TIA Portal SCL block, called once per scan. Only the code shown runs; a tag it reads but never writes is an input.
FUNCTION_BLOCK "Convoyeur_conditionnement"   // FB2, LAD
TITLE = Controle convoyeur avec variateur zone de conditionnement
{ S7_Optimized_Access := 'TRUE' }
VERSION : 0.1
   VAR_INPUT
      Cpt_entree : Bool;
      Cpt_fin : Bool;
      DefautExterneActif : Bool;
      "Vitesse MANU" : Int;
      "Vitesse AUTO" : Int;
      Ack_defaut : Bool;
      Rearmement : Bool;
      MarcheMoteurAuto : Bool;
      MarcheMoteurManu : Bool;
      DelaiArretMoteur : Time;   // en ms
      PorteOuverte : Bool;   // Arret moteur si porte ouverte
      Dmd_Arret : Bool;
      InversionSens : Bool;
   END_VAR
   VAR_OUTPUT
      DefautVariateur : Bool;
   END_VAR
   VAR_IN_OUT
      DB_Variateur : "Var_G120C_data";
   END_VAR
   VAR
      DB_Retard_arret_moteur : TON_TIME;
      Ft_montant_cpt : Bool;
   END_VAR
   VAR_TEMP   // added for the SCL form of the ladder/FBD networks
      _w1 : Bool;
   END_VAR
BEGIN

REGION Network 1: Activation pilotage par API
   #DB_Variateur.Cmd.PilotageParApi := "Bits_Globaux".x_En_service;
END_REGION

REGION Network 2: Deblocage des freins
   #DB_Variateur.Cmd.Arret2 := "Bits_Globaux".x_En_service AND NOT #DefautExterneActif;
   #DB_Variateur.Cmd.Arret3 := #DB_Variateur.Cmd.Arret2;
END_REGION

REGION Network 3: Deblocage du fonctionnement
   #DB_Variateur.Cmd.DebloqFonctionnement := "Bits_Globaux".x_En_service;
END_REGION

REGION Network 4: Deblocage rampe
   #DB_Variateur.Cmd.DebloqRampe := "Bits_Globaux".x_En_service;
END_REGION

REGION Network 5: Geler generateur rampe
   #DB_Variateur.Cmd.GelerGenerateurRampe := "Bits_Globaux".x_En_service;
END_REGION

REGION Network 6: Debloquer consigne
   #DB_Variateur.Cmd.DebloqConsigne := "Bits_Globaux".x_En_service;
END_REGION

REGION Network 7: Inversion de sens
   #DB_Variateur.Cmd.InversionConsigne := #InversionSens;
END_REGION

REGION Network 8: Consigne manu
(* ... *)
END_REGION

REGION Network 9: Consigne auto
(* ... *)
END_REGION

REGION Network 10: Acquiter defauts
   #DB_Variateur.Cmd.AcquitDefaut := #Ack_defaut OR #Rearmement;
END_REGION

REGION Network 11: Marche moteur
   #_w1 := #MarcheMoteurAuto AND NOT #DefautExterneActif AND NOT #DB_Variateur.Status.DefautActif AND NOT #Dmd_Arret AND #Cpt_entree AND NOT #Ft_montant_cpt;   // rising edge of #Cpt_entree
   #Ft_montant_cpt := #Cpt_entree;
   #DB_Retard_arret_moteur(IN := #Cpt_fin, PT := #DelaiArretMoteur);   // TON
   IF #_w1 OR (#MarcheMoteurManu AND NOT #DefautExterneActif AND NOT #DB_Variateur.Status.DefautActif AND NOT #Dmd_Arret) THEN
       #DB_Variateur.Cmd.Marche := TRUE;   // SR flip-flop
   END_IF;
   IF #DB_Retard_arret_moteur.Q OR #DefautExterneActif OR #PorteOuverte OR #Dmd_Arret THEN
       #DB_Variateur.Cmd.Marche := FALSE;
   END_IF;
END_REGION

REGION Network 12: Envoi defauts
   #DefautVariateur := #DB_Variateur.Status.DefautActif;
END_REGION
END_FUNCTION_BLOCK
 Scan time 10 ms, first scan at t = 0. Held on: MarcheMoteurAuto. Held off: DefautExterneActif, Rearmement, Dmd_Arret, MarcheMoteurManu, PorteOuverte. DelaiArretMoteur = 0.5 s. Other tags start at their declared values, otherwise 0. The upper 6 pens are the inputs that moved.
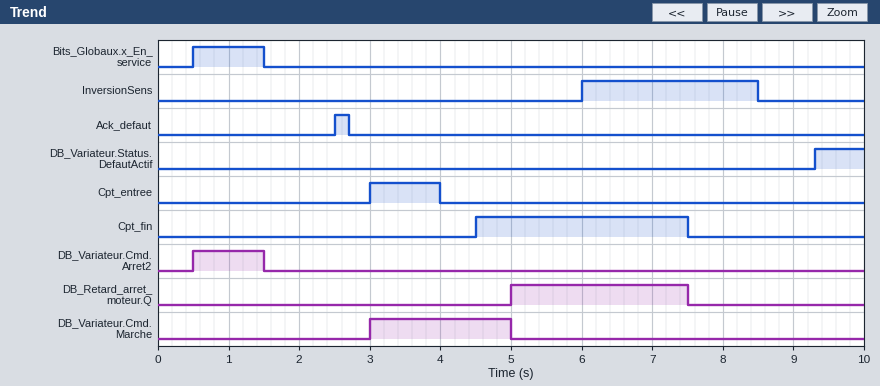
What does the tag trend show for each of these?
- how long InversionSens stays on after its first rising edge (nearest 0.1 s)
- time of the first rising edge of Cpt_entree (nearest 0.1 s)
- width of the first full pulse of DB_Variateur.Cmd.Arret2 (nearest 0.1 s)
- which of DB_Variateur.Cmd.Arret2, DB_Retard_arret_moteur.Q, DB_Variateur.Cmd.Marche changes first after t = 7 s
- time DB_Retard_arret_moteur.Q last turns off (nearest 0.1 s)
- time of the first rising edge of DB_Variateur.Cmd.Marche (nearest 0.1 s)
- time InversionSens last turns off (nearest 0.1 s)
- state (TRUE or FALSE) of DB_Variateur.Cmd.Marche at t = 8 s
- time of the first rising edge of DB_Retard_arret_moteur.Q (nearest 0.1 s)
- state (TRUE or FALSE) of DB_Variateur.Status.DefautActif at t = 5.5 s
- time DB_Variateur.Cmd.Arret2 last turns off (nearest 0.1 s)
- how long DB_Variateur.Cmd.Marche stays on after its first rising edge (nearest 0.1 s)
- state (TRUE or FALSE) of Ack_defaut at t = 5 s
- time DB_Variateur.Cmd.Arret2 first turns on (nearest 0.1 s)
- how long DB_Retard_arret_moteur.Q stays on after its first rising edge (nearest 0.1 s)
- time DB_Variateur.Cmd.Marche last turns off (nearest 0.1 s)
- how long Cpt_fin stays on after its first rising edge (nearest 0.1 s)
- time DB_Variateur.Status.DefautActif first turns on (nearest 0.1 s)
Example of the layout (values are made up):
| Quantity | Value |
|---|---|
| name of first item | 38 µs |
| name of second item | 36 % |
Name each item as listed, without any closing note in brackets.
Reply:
| Quantity | Value |
|---|---|
| how long InversionSens stays on after its first rising edge | 2.5 s |
| time of the first rising edge of Cpt_entree | 3.0 s |
| width of the first full pulse of DB_Variateur.Cmd.Arret2 | 1.0 s |
| which of DB_Variateur.Cmd.Arret2, DB_Retard_arret_moteur.Q, DB_Variateur.Cmd.Marche changes first after t = 7 s | DB_Retard_arret_moteur.Q |
| time DB_Retard_arret_moteur.Q last turns off | 7.5 s |
| time of the first rising edge of DB_Variateur.Cmd.Marche | 3.0 s |
| time InversionSens last turns off | 8.5 s |
| state (TRUE or FALSE) of DB_Variateur.Cmd.Marche at t = 8 s | FALSE |
| time of the first rising edge of DB_Retard_arret_moteur.Q | 5.0 s |
| state (TRUE or FALSE) of DB_Variateur.Status.DefautActif at t = 5.5 s | FALSE |
| time DB_Variateur.Cmd.Arret2 last turns off | 1.5 s |
| how long DB_Variateur.Cmd.Marche stays on after its first rising edge | 2.0 s |
| state (TRUE or FALSE) of Ack_defaut at t = 5 s | FALSE |
| time DB_Variateur.Cmd.Arret2 first turns on | 0.5 s |
| how long DB_Retard_arret_moteur.Q stays on after its first rising edge | 2.5 s |
| time DB_Variateur.Cmd.Marche last turns off | 5.0 s |
| how long Cpt_fin stays on after its first rising edge | 3.0 s |
| time DB_Variateur.Status.DefautActif first turns on | 9.3 s |
